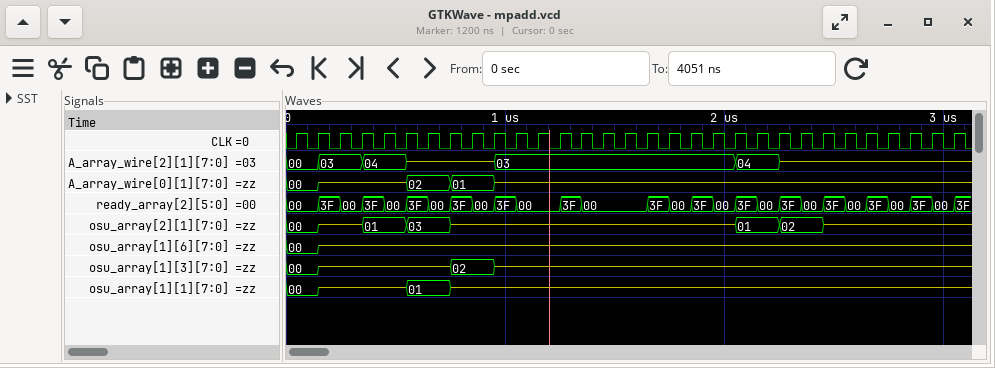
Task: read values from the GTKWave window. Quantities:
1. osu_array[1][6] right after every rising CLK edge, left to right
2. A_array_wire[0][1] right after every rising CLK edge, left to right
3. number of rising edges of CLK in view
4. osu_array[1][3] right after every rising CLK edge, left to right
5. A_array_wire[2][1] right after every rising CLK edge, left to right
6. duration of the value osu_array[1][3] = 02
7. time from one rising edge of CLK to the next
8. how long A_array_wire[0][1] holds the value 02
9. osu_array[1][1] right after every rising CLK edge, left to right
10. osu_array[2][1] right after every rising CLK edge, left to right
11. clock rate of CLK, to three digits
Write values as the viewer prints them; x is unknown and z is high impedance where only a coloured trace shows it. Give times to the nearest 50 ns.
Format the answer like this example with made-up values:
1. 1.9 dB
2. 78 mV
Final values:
1. 00, z, z, z, z, z, z, z, z, z, z, z, z, z, z, z, z, z, z, z, z, z, z, z, z, z, z, z, z, z, z
2. 00, z, z, z, z, 02, 02, 01, 01, z, z, z, z, z, z, z, z, z, z, z, z, z, z, z, z, z, z, z, z, z, z
3. 31
4. 00, z, z, z, z, z, z, 02, 02, z, z, z, z, z, z, z, z, z, z, z, z, z, z, z, z, z, z, z, z, z, z
5. 00, 03, 03, 04, 04, z, z, z, z, 03, 03, 03, 03, 03, 03, 03, 03, 03, 03, 03, 04, 04, z, z, z, z, z, z, z, z, z
6. 200 ns
7. 100 ns
8. 200 ns
9. 00, z, z, z, z, 01, 01, z, z, z, z, z, z, z, z, z, z, z, z, z, z, z, z, z, z, z, z, z, z, z, z
10. 00, z, z, 01, 01, 03, 03, z, z, z, z, z, z, z, z, z, z, z, z, z, 01, 01, 02, 02, z, z, z, z, z, z, z
11. 10.0 MHz
